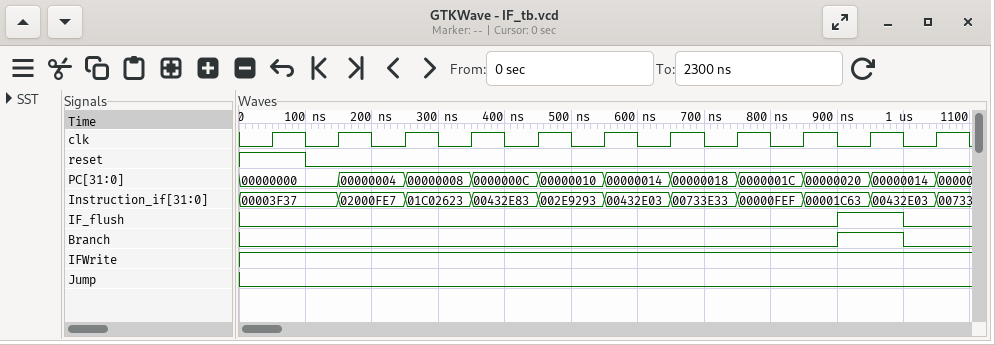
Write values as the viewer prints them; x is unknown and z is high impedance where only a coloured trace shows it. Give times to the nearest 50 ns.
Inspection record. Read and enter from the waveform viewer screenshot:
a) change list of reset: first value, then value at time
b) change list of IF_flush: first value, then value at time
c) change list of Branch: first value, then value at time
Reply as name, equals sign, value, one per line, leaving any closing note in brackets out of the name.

change list of reset: first value, then value at time = 1, 0 at 100 ns
change list of IF_flush: first value, then value at time = 0, 1 at 900 ns, 0 at 1000 ns
change list of Branch: first value, then value at time = 0, 1 at 900 ns, 0 at 1000 ns
